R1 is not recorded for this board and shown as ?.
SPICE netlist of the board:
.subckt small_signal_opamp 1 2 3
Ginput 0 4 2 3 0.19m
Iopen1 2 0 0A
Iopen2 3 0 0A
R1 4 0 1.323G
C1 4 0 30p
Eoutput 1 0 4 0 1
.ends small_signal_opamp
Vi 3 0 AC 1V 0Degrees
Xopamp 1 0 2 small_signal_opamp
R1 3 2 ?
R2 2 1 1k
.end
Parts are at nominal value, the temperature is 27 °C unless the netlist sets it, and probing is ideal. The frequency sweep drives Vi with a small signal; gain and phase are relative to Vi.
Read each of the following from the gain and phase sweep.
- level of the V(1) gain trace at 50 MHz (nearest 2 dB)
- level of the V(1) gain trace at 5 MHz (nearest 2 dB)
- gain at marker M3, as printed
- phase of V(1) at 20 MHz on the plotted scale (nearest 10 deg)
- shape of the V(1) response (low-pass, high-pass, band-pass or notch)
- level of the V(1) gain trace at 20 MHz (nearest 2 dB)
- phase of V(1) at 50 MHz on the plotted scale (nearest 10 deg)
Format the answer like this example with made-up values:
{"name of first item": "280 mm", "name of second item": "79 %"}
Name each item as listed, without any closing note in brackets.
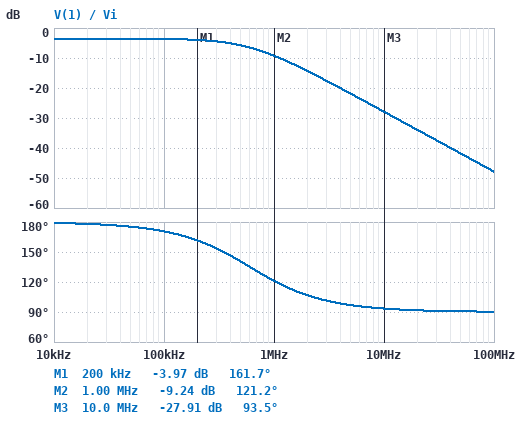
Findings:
{"level of the V(1) gain trace at 50 MHz": "-42 dB", "level of the V(1) gain trace at 5 MHz": "-22 dB", "gain at marker M3, as printed": "-27.91 dB", "phase of V(1) at 20 MHz on the plotted scale": "90 deg", "shape of the V(1) response": "low-pass", "level of the V(1) gain trace at 20 MHz": "-34 dB", "phase of V(1) at 50 MHz on the plotted scale": "90 deg"}
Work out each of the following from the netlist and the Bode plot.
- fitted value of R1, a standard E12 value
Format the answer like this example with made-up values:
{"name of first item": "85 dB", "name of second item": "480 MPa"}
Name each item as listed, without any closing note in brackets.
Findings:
{"fitted value of R1, a standard E12 value": "1.5 kΩ"}
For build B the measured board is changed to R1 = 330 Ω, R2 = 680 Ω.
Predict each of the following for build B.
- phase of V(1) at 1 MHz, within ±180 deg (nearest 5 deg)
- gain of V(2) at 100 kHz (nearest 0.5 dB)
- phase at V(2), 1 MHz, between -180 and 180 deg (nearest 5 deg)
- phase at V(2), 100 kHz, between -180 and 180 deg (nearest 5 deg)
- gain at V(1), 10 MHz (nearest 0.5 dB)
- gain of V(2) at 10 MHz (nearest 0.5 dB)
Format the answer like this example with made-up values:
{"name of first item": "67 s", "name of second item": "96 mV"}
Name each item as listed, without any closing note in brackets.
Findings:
{"phase of V(1) at 1 MHz, within ±180 deg": "110 deg", "gain of V(2) at 100 kHz": "-14.0 dB", "phase at V(2), 1 MHz, between -180 and 180 deg": "20 deg", "phase at V(2), 100 kHz, between -180 and 180 deg": "75 deg", "gain at V(1), 10 MHz": "-23.5 dB", "gain of V(2) at 10 MHz": "-3.5 dB"}
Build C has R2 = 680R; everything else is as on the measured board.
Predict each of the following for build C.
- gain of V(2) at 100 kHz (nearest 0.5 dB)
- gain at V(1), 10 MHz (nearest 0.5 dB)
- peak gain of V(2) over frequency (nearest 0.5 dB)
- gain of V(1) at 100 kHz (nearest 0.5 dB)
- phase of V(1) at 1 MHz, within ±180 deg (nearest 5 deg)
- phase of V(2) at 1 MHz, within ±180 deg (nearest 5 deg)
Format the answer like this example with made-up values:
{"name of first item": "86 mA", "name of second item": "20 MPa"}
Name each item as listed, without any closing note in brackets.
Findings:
{"gain of V(2) at 100 kHz": "-27.0 dB", "gain at V(1), 10 MHz": "-30.0 dB", "peak gain of V(2) over frequency": "-10.0 dB", "gain of V(1) at 100 kHz": "-7.0 dB", "phase of V(1) at 1 MHz, within ±180 deg": "125 deg", "phase of V(2) at 1 MHz, within ±180 deg": "35 deg"}
